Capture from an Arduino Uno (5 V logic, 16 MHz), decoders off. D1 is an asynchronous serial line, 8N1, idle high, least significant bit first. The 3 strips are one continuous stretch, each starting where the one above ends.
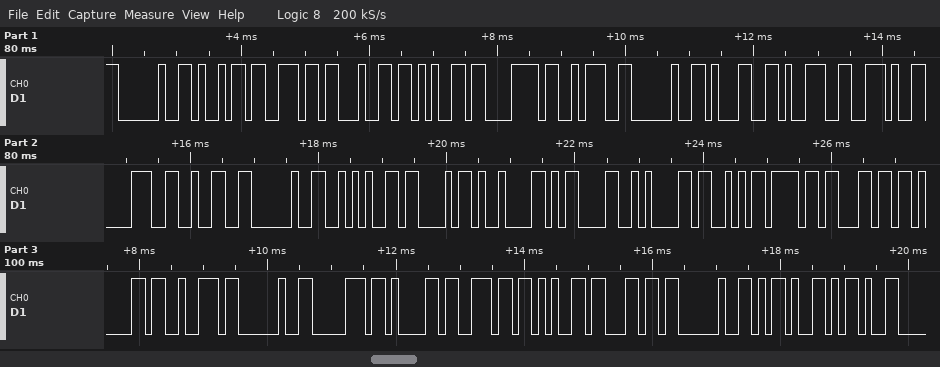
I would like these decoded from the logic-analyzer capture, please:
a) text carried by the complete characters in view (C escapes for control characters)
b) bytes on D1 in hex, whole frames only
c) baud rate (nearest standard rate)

" index: 19.82 *C\t\r\nSolar panel --"
20 69 6E 64 65 78 3A 20 31 39 2E 38 32 20 2A 43 09 0D 0A 53 6F 6C 61 72 20 70 61 6E 65 6C 20 2D 2D
9600 baud
